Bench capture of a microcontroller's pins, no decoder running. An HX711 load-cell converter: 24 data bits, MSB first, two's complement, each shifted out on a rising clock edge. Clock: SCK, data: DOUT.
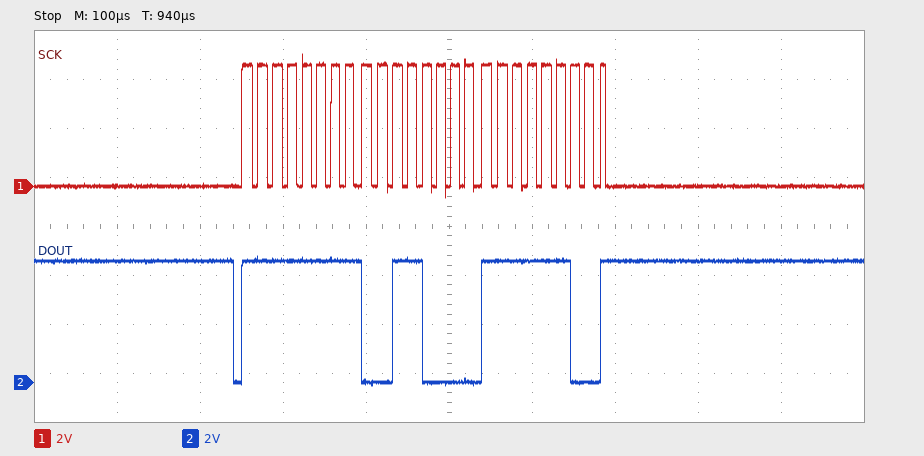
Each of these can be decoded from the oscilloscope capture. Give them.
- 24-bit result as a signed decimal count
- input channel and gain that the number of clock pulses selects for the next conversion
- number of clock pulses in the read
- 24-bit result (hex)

-52996
channel A, gain 128
25
0xFF30FC
